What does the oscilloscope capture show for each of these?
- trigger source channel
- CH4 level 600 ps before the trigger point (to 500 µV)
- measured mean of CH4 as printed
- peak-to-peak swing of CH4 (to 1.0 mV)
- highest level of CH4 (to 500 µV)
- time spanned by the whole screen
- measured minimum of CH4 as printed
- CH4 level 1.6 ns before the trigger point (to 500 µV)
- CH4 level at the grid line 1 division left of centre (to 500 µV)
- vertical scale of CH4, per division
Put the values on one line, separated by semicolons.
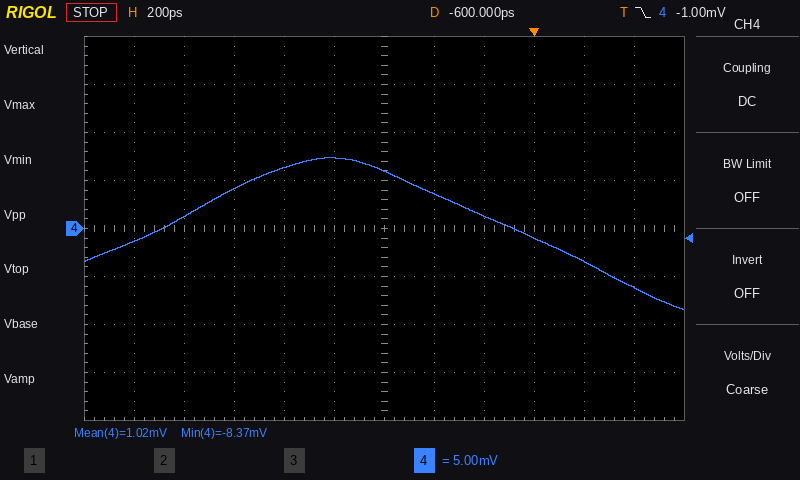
CH4; 6.0 mV; 1.02 mV; 16.0 mV; 7.5 mV; 2.4 ns; -8.37 mV; -1.5 mV; 7.5 mV; 5 mV
